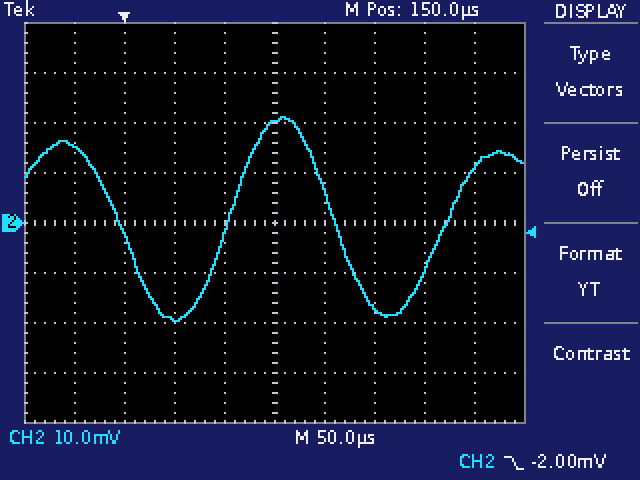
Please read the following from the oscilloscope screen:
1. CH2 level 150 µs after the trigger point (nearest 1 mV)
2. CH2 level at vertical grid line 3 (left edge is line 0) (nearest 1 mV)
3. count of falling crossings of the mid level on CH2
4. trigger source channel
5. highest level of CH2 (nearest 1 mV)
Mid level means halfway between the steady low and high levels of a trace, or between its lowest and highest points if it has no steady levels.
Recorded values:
20 mV
-19 mV
2
CH2
21 mV
